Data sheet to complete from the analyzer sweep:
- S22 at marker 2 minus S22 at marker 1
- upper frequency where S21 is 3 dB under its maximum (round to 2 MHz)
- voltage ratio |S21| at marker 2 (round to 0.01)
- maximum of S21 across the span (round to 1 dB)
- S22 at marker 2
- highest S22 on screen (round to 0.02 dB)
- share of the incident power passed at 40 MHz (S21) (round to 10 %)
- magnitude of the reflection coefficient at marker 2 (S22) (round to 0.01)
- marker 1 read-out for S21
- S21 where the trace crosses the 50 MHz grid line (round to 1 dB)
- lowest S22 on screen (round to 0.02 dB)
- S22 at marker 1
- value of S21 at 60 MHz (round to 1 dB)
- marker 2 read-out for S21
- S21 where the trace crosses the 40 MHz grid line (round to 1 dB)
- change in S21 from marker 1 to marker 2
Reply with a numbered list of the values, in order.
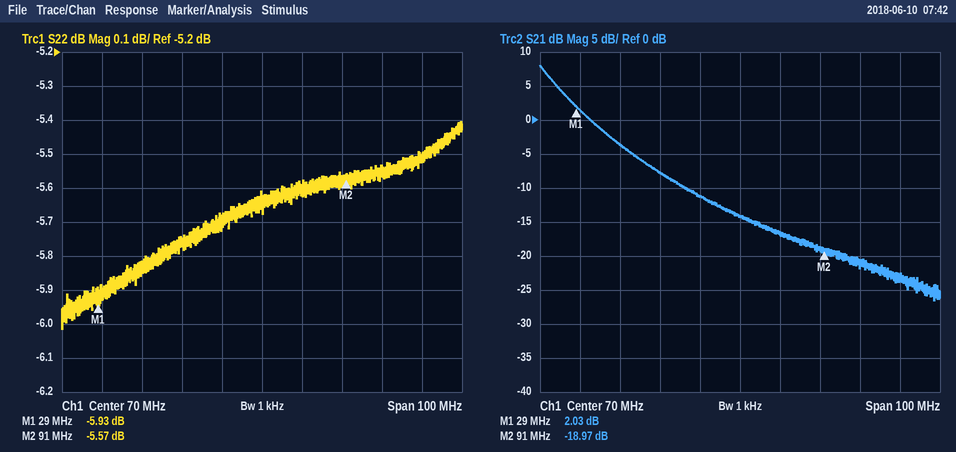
1. 0.36 dB
2. 24 MHz
3. 0.11
4. 8 dB
5. -5.57 dB
6. -5.40 dB
7. 40 %
8. 0.53
9. 2.03 dB
10. -8 dB
11. -6.02 dB
12. -5.93 dB
13. -11 dB
14. -18.97 dB
15. -4 dB
16. -21.00 dB
